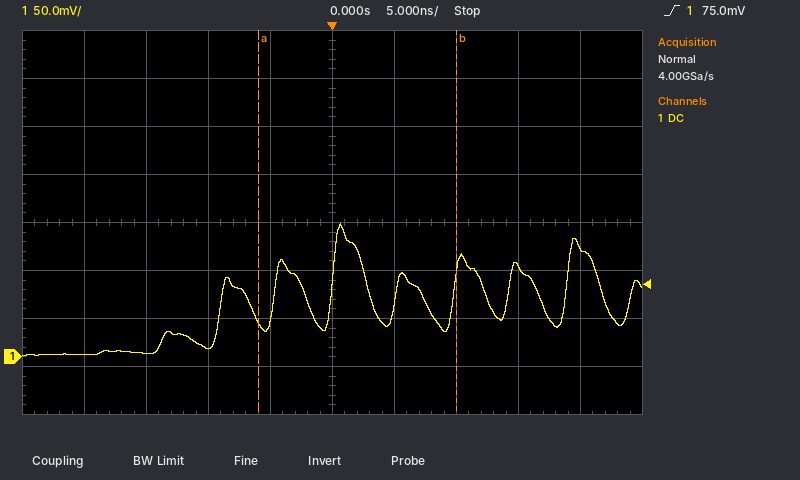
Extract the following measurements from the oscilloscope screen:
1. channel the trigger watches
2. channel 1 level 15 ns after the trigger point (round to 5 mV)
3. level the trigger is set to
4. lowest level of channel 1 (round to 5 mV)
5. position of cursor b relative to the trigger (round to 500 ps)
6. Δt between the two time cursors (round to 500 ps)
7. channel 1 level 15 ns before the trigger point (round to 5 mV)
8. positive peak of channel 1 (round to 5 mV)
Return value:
channel 1
95 mV
75.0 mV
0 mV
+10.0 ns
16.0 ns
5 mV
140 mV
